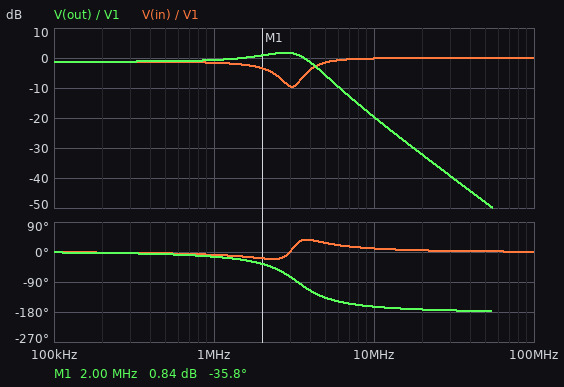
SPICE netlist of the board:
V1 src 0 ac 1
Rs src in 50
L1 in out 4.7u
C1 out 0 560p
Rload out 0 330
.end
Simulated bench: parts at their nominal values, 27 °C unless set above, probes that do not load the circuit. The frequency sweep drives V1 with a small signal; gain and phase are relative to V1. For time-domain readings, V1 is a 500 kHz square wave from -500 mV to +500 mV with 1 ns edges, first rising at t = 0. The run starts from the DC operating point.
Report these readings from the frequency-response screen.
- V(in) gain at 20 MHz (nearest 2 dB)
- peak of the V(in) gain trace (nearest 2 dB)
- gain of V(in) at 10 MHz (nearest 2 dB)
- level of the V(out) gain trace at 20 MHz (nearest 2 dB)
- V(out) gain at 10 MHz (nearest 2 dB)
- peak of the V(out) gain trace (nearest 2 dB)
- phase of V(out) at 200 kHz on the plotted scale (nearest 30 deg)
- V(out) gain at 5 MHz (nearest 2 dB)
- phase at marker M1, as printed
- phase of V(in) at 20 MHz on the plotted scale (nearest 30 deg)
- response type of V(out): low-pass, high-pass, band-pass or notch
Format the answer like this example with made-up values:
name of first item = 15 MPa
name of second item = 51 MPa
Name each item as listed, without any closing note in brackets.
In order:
V(in) gain at 20 MHz = 0 dB
peak of the V(in) gain trace = 0 dB
gain of V(in) at 10 MHz = 0 dB
level of the V(out) gain trace at 20 MHz = -32 dB
V(out) gain at 10 MHz = -20 dB
peak of the V(out) gain trace = 2 dB
phase of V(out) at 200 kHz on the plotted scale = 0 deg
V(out) gain at 5 MHz = -6 dB
phase at marker M1, as printed = -35.8 deg
phase of V(in) at 20 MHz on the plotted scale = 0 deg
response type of V(out): low-pass, high-pass, band-pass or notch = low-pass
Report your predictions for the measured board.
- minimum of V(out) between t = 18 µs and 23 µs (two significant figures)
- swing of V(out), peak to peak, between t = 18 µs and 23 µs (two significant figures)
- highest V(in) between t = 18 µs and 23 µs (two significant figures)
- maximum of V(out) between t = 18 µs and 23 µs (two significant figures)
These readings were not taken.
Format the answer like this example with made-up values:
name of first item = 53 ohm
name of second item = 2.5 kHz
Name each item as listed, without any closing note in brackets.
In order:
minimum of V(out) between t = 18 µs and 23 µs = -670 mV
swing of V(out), peak to peak, between t = 18 µs and 23 µs = 1.3 V
highest V(in) between t = 18 µs and 23 µs = 560 mV
maximum of V(out) between t = 18 µs and 23 µs = 670 mV
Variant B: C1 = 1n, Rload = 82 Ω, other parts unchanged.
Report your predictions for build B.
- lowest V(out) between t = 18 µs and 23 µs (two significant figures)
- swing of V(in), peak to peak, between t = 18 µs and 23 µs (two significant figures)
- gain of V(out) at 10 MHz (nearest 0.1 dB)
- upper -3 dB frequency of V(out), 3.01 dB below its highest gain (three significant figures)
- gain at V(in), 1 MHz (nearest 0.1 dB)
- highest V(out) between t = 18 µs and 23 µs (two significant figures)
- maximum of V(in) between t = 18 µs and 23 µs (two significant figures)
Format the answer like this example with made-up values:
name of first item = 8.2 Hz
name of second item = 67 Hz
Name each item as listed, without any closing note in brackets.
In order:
lowest V(out) between t = 18 µs and 23 µs = -360 mV
swing of V(in), peak to peak, between t = 18 µs and 23 µs = 1.4 V
gain of V(out) at 10 MHz = -25.2 dB
upper -3 dB frequency of V(out), 3.01 dB below its highest gain = 3.24 MHz
gain at V(in), 1 MHz = -5.0 dB
highest V(out) between t = 18 µs and 23 µs = 360 mV
maximum of V(in) between t = 18 µs and 23 µs = 680 mV
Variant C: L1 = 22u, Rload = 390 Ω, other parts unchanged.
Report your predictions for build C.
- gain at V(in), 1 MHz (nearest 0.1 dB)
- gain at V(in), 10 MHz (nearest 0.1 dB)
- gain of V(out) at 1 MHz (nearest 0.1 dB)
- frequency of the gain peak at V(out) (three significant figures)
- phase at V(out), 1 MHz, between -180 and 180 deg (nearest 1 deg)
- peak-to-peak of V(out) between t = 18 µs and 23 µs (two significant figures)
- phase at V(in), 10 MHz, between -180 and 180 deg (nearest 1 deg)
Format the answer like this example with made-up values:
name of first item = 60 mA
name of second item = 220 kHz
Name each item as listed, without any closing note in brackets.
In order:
gain at V(in), 1 MHz = -2.5 dB
gain at V(in), 10 MHz = 0 dB
gain of V(out) at 1 MHz = 1.6 dB
frequency of the gain peak at V(out) = 1.31 MHz
phase at V(out), 1 MHz, between -180 and 180 deg = -40 deg
peak-to-peak of V(out) between t = 18 µs and 23 µs = 1.4 V
phase at V(in), 10 MHz, between -180 and 180 deg = 2 deg
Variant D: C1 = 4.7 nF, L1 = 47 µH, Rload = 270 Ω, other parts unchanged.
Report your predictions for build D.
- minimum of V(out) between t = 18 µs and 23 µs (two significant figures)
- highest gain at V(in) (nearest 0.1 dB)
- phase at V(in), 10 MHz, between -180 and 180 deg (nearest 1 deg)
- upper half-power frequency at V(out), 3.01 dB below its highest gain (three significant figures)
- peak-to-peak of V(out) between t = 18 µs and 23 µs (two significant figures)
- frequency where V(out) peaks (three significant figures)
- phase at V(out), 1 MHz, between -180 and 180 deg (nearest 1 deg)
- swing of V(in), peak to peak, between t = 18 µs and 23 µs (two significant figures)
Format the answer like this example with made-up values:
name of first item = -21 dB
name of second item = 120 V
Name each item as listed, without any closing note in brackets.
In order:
minimum of V(out) between t = 18 µs and 23 µs = -400 mV
highest gain at V(in) = 0 dB
phase at V(in), 10 MHz, between -180 and 180 deg = 1 deg
upper half-power frequency at V(out), 3.01 dB below its highest gain = 438 kHz
peak-to-peak of V(out) between t = 18 µs and 23 µs = 800 mV
frequency where V(out) peaks = 304 kHz
phase at V(out), 1 MHz, between -180 and 180 deg = -161 deg
swing of V(in), peak to peak, between t = 18 µs and 23 µs = 1.6 V
